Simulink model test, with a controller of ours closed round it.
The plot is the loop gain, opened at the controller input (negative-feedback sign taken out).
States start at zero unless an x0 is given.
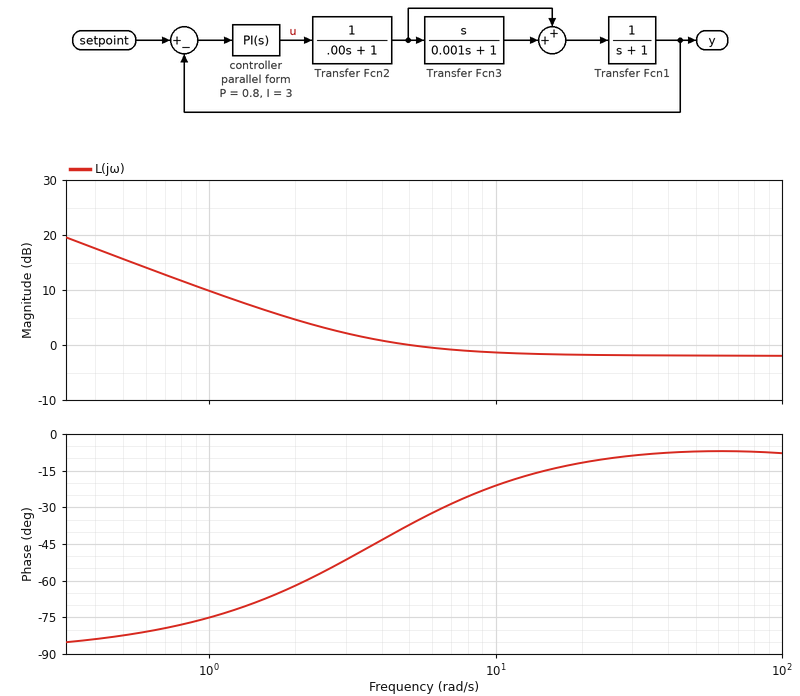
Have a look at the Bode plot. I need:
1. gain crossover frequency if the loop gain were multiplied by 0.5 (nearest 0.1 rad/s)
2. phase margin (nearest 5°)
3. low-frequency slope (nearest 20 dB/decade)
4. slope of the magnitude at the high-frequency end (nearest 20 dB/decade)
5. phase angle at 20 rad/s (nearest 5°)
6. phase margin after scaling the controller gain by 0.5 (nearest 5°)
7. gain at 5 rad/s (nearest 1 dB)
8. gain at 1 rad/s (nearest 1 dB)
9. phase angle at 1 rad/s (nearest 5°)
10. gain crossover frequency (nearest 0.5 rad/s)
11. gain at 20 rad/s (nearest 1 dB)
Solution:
1.6 rad/s
145°
-20 dB/decade
0 dB/decade
-10°
115°
0 dB
10 dB
-75°
5.0 rad/s
-2 dB
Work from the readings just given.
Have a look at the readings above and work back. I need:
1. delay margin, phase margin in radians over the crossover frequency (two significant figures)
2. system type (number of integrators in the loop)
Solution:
0.51 s
1
